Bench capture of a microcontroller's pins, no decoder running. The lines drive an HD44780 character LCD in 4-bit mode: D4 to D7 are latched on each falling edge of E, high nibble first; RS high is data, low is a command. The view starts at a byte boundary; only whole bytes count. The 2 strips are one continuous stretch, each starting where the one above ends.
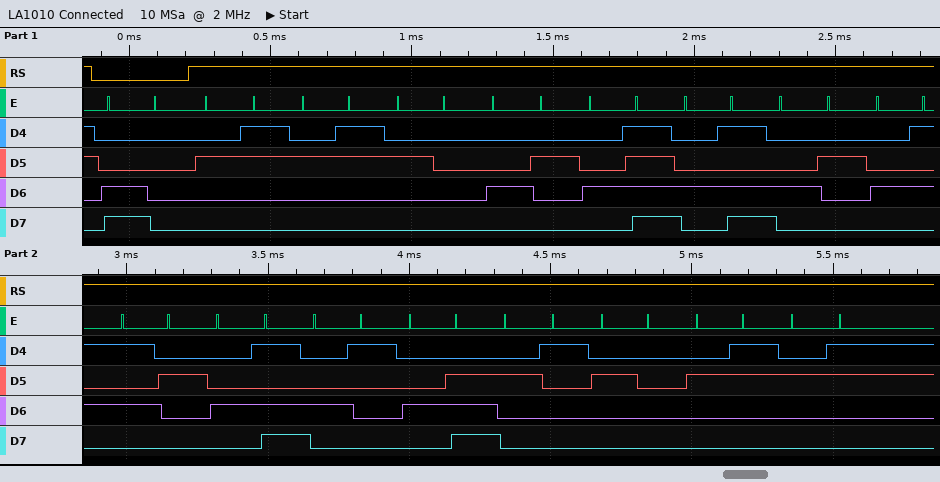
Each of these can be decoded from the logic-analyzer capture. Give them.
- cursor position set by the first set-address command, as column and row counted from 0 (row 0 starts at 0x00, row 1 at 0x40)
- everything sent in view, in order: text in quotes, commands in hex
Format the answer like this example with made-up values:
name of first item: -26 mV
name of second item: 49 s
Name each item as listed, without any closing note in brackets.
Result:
cursor position set by the first set-address command, as column and row counted from 0: column 0, row 1
everything sent in view, in order: text in quotes, commands in hex: 0xC0 "## BOMBERMAN! ##"
